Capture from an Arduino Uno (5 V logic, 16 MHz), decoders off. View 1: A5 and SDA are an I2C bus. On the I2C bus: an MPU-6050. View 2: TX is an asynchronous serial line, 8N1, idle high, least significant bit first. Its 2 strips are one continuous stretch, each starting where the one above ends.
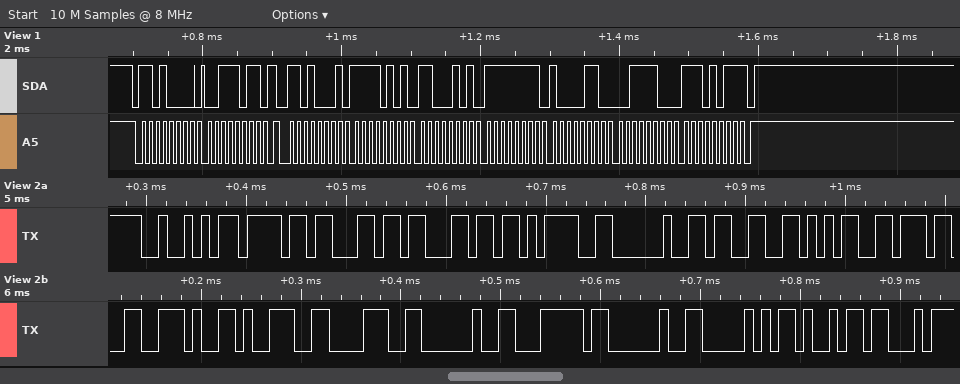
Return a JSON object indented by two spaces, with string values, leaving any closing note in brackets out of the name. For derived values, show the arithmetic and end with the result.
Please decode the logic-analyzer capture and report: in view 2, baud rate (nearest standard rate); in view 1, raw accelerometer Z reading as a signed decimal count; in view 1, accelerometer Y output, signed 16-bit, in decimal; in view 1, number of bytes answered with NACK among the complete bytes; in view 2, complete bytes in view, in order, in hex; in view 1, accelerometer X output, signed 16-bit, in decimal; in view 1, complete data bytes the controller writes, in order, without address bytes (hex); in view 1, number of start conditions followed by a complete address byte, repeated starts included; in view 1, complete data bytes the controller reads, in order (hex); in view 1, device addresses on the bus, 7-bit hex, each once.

{
  "in view 2, baud rate": "115200 baud",
  "in view 1, raw accelerometer Z reading as a signed decimal count": "0x3CEB = 15595",
  "in view 1, accelerometer Y output, signed 16-bit, in decimal": "0xFF86 = -122",
  "in view 1, number of bytes answered with NACK among the complete bytes": "1",
  "in view 2, complete bytes in view, in order, in hex": "0x52 0x6F 0x6C 0x6C 0x3D 0x20 0x33 0x35 0x37 0x2E 0x39 0x38 0x20 0x7C 0x20 0x50 0x69",
  "in view 1, accelerometer X output, signed 16-bit, in decimal": "0xF5C5 = -2619",
  "in view 1, complete data bytes the controller writes, in order, without address bytes": "3B",
  "in view 1, number of start conditions followed by a complete address byte, repeated starts included": "2",
  "in view 1, complete data bytes the controller reads, in order": "F5 C5 FF 86 3C EB",
  "in view 1, device addresses on the bus, 7-bit hex, each once": "0x68"
}
